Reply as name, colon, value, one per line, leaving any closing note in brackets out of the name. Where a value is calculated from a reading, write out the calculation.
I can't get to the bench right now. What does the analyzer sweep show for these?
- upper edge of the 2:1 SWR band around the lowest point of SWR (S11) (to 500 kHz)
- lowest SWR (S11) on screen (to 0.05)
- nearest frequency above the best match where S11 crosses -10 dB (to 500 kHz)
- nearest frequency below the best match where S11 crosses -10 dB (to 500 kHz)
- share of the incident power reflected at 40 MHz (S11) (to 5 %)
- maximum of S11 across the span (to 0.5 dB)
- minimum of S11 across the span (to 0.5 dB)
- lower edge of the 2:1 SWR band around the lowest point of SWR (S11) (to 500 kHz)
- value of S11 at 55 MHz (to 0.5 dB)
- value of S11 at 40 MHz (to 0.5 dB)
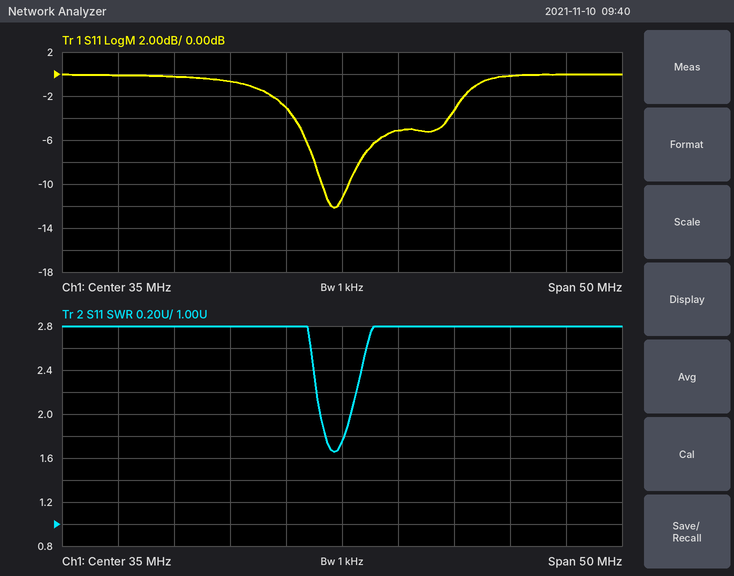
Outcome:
upper edge of the 2:1 SWR band around the lowest point of SWR (S11): 36.0 MHz
lowest SWR (S11) on screen: 1.65
nearest frequency above the best match where S11 crosses -10 dB: 35.5 MHz
nearest frequency below the best match where S11 crosses -10 dB: 33.0 MHz
share of the incident power reflected at 40 MHz (S11): 10^(-5/10) ≈ 31.6 %, so 30 % to the nearest 5 %
maximum of S11 across the span: 0.0 dB
minimum of S11 across the span: -12.0 dB
lower edge of the 2:1 SWR band around the lowest point of SWR (S11): 33.0 MHz
value of S11 at 55 MHz: 0.0 dB
value of S11 at 40 MHz: -5.0 dB
